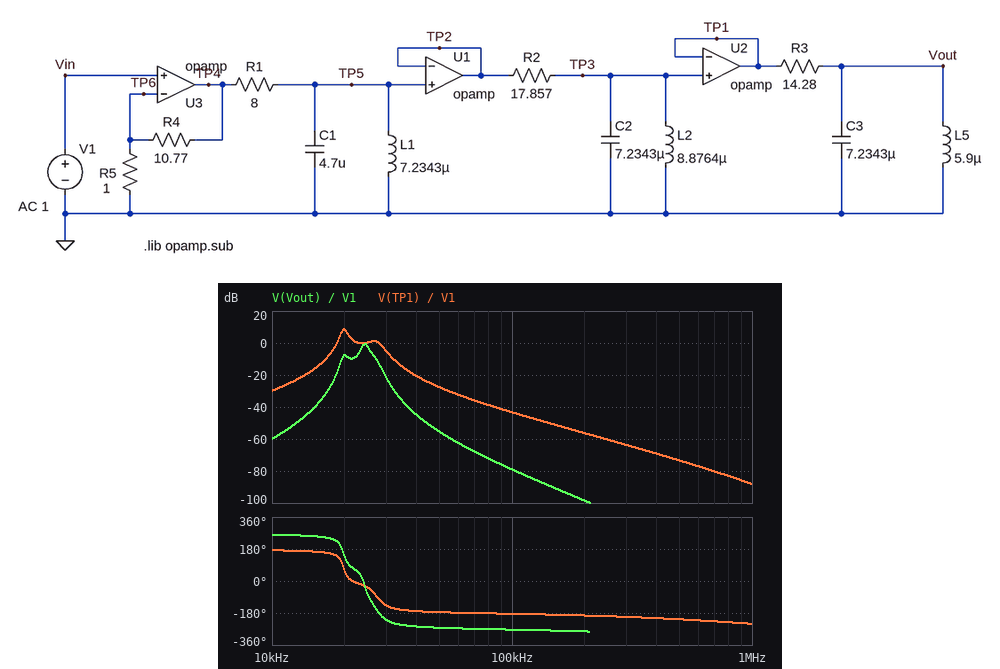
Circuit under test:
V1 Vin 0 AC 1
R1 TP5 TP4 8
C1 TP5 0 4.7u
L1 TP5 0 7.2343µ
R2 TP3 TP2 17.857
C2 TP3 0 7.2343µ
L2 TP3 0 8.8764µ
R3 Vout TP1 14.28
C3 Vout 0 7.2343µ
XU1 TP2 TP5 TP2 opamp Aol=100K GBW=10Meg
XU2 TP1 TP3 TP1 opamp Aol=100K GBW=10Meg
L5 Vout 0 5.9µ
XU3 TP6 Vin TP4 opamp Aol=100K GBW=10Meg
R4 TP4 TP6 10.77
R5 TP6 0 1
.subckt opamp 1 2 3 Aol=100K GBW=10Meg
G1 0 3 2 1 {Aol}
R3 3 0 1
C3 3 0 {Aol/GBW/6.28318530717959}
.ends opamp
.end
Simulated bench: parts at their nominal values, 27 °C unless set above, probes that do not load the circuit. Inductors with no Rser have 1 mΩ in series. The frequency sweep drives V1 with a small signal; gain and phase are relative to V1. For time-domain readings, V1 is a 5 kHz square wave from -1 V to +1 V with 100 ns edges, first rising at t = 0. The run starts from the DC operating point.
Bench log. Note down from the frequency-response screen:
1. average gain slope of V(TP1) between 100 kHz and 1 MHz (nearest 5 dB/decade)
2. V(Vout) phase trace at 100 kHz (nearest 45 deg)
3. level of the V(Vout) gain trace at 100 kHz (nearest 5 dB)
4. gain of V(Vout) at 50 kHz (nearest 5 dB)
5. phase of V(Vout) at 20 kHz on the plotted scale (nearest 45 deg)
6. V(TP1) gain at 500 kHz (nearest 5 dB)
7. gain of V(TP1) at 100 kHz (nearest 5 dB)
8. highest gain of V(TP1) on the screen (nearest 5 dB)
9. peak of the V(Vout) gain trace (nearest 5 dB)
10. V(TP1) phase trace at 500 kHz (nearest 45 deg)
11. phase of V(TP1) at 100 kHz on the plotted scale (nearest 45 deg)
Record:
-45 dB/decade
-270 deg
-80 dB
-55 dB
135 deg
-75 dB
-45 dB
10 dB
0 dB
-225 deg
-180 deg
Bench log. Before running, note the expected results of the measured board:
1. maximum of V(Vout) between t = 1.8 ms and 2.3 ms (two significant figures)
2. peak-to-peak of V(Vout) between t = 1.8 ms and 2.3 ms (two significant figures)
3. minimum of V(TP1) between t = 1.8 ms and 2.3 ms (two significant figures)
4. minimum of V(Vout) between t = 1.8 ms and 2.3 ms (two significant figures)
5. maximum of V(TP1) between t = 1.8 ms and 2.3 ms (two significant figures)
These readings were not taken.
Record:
200 mV
400 mV
-330 mV
-200 mV
330 mV
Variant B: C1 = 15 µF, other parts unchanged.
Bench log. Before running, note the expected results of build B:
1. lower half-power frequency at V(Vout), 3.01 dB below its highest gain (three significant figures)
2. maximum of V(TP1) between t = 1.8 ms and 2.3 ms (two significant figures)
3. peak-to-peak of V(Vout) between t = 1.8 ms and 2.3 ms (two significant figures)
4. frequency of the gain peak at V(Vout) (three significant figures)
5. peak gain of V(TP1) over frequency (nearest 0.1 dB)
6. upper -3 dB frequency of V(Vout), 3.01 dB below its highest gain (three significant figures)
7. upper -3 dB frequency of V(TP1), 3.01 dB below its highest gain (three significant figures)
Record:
19.3 kHz
510 mV
110 mV
19.9 kHz
5.5 dB
20.6 kHz
20.4 kHz
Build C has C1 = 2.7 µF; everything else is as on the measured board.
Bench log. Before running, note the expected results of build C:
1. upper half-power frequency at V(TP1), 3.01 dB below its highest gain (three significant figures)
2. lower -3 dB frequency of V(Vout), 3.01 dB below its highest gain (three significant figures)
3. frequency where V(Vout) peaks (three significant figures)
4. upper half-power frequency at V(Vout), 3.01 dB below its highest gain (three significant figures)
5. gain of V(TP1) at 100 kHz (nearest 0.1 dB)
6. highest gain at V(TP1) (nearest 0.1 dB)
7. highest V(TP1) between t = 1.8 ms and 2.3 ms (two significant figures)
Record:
20.6 kHz
23.4 kHz
24.3 kHz
25.1 kHz
-38.0 dB
5.4 dB
260 mV
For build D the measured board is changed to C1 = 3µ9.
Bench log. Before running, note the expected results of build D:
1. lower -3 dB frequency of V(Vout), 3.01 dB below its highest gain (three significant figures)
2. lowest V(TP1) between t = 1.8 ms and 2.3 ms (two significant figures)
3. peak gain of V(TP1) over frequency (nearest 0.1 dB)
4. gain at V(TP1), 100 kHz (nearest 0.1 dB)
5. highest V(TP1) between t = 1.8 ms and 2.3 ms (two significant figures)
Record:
23.5 kHz
-250 mV
7.2 dB
-41.5 dB
250 mV
